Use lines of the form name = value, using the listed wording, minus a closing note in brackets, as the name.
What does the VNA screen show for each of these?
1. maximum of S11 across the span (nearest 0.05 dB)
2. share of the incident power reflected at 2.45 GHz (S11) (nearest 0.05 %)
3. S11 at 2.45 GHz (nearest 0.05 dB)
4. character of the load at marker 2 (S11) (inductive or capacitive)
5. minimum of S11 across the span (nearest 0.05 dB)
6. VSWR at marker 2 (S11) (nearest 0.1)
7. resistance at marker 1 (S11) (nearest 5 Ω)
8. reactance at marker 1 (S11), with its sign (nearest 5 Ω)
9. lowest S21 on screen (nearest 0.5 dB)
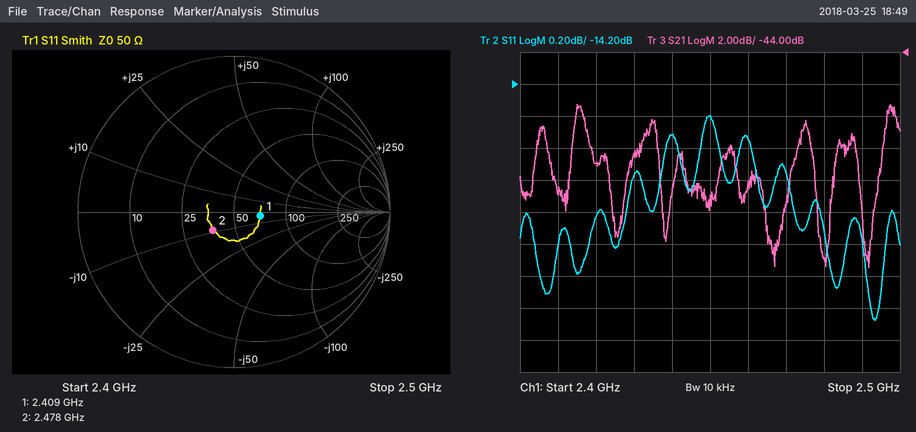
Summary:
maximum of S11 across the span = -14.40 dB
share of the incident power reflected at 2.45 GHz (S11) = 3.65 %
S11 at 2.45 GHz = -14.40 dB
character of the load at marker 2 (S11) = capacitive
minimum of S11 across the span = -15.70 dB
VSWR at marker 2 (S11) = 1.4
resistance at marker 1 (S11) = 70 Ω
reactance at marker 1 (S11), with its sign = -5 Ω
lowest S21 on screen = -57.5 dB
